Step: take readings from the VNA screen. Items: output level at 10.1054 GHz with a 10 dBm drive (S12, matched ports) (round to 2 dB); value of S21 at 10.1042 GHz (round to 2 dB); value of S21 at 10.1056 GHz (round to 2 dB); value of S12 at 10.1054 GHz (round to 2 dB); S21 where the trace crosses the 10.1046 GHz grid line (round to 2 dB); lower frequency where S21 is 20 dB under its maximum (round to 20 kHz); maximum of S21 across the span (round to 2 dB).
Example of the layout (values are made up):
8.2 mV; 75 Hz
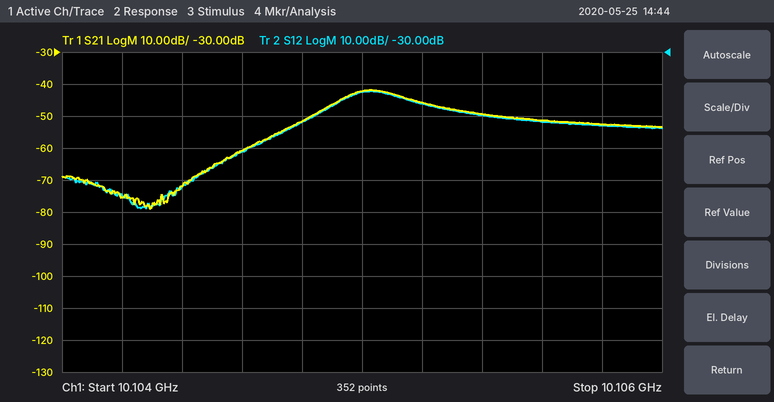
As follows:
-40 dBm; -76 dB; -52 dB; -50 dB; -60 dB; 10.10458 GHz; -42 dB
